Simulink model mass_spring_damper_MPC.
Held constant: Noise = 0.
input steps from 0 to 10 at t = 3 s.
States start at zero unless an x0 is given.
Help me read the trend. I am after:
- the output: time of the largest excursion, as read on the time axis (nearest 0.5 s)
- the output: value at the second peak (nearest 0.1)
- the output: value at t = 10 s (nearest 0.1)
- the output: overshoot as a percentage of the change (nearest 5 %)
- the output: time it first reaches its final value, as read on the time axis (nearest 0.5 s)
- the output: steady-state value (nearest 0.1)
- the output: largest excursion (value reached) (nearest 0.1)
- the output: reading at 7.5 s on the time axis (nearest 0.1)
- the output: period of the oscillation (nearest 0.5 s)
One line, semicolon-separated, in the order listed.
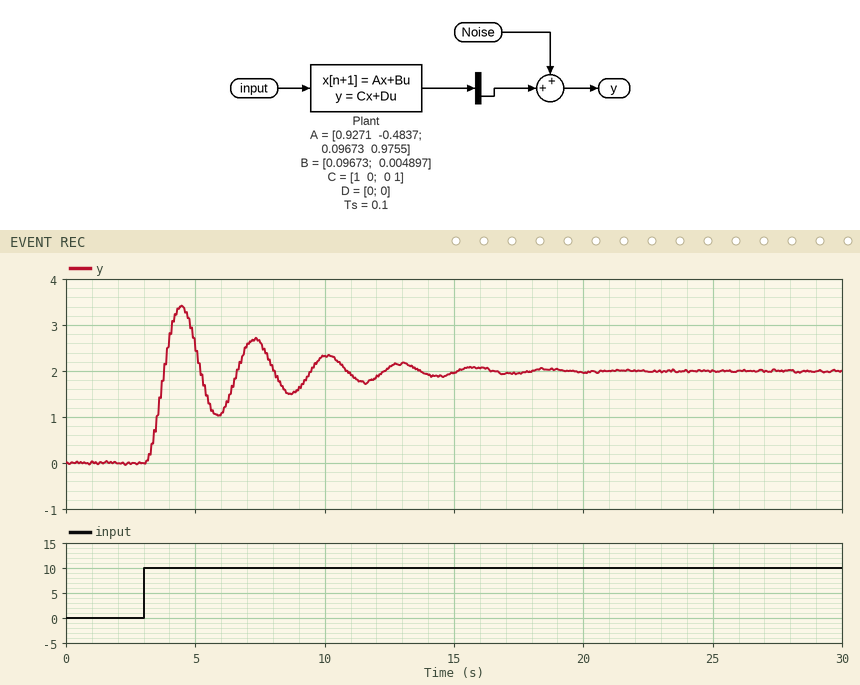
4.5 s; 2.7; 2.3; 70 %; 4.0 s; 2.0; 3.4; 2.6; 3.0 s
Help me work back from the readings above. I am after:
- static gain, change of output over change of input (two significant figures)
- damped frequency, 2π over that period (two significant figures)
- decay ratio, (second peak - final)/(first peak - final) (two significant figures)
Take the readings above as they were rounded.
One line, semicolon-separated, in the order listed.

0.20; 2.1 rad/s; 0.50
